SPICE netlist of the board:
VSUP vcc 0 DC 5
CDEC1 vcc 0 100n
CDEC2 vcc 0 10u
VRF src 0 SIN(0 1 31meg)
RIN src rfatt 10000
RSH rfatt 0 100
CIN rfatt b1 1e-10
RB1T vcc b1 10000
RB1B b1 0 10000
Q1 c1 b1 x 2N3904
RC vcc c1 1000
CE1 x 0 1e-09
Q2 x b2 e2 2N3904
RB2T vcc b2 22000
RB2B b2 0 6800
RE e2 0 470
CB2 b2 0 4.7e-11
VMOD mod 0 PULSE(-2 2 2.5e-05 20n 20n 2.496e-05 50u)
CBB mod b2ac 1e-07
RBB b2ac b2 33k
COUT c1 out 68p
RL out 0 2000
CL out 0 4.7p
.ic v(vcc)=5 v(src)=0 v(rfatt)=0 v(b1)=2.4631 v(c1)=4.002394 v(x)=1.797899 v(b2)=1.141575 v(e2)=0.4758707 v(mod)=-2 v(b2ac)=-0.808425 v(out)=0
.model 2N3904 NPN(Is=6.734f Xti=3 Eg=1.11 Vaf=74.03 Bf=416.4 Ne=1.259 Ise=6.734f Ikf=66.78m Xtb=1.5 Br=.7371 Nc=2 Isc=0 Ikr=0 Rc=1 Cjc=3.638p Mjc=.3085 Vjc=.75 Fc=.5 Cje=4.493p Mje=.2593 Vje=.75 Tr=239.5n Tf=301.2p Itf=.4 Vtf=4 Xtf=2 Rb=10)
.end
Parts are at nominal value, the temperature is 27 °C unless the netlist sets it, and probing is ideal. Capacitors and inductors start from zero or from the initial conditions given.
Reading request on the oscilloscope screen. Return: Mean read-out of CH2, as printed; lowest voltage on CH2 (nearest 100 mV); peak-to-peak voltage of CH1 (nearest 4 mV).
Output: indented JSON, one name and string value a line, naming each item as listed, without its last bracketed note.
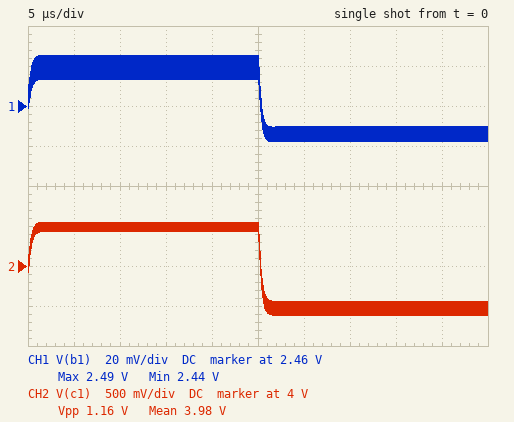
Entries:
{
  "Mean read-out of CH2, as printed": "3.98 V",
  "lowest voltage on CH2": "3.4 V",
  "peak-to-peak voltage of CH1": "44 mV"
}
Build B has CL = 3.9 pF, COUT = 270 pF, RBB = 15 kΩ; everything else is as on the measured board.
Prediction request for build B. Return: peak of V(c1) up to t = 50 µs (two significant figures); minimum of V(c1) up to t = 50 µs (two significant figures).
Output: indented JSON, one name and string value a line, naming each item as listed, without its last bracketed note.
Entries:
{
  "peak of V(c1) up to t = 50 µs": "4.9 V",
  "minimum of V(c1) up to t = 50 µs": "2.9 V"
}
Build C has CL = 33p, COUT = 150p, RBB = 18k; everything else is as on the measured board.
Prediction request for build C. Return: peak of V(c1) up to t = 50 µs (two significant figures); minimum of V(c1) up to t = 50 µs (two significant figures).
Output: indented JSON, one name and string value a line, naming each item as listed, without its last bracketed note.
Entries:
{
  "peak of V(c1) up to t = 50 µs": "4.8 V",
  "minimum of V(c1) up to t = 50 µs": "3.1 V"
}
